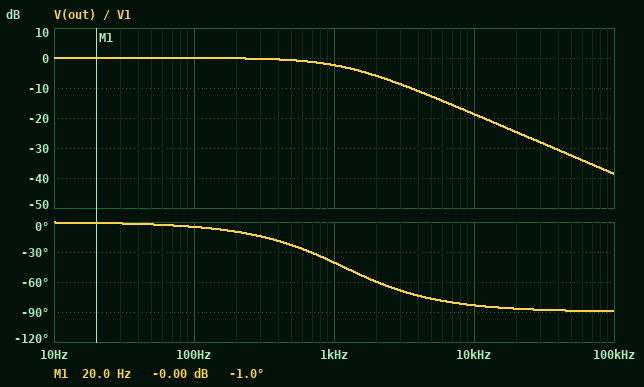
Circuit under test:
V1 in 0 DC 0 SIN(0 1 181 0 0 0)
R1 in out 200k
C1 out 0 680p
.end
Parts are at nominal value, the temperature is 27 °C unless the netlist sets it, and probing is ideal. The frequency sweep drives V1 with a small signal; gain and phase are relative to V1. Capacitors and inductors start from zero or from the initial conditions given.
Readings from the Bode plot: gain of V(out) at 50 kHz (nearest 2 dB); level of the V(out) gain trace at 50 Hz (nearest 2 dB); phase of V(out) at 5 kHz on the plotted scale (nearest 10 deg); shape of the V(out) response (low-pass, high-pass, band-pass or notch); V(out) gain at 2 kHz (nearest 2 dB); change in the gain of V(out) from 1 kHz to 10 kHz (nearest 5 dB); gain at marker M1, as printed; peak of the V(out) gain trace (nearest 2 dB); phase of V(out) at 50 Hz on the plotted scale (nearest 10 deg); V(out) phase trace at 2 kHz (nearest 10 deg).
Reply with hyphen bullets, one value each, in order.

- -32 dB
- 0 dB
- -80 deg
- low-pass
- -6 dB
- -15 dB
- -0.00 dB
- 0 dB
- 0 deg
- -60 deg
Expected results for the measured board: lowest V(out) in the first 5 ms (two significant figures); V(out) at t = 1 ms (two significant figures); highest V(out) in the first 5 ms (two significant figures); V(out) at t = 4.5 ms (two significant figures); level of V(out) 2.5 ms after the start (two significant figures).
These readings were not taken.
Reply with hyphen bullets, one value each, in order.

- -990 mV
- 820 mV
- 990 mV
- -960 mV
- 430 mV
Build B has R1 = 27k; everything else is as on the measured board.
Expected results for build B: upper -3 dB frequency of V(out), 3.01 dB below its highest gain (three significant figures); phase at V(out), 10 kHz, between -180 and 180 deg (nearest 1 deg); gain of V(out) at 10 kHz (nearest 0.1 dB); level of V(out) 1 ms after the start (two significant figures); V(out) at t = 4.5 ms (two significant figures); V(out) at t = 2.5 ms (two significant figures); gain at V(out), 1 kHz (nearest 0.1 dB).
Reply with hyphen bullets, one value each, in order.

- 8.67 kHz
- -49 deg
- -3.7 dB
- 900 mV
- -930 mV
- 310 mV
- -0.1 dB
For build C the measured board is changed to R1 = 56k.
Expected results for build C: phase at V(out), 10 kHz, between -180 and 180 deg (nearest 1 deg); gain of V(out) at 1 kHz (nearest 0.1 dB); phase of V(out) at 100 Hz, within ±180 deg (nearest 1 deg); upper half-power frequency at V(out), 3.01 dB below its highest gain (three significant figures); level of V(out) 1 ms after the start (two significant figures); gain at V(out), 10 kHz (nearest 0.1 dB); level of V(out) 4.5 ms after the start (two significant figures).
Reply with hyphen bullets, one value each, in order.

- -67 deg
- -0.2 dB
- -1 deg
- 4.18 kHz
- 890 mV
- -8.3 dB
- -930 mV
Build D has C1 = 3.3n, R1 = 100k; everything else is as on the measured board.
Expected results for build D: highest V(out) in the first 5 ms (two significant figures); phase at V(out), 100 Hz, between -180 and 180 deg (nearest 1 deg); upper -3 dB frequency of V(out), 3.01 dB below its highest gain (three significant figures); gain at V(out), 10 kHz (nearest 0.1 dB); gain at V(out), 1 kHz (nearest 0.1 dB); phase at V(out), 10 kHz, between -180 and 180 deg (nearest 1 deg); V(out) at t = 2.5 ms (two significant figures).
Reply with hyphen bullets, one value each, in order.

- 940 mV
- -12 deg
- 482 Hz
- -26.3 dB
- -7.2 dB
- -87 deg
- 570 mV
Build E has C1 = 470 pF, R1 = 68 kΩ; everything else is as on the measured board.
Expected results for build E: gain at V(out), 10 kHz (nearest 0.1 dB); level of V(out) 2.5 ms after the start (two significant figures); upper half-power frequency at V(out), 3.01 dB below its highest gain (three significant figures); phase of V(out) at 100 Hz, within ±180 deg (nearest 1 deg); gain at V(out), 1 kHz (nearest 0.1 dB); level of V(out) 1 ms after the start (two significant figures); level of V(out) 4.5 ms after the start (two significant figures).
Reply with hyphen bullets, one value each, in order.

- -7.0 dB
- 330 mV
- 4.98 kHz
- -1 deg
- -0.2 dB
- 890 mV
- -930 mV
